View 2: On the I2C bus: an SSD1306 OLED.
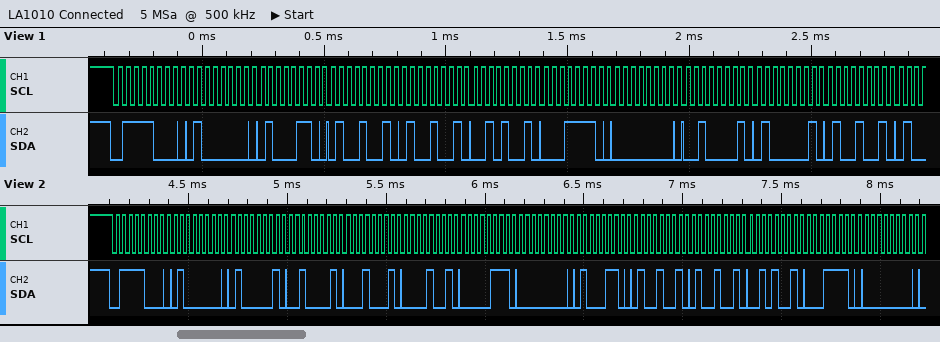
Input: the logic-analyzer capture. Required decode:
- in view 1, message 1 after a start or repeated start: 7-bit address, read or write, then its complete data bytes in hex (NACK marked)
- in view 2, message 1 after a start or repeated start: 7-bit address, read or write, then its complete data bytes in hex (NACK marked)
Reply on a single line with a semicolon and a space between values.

0x3C write: 40 46 49 49 29 1E 00 21 41 49; 0x3C write: 40 41 21 11 09 07 00 46 49 49 29 1E 00
